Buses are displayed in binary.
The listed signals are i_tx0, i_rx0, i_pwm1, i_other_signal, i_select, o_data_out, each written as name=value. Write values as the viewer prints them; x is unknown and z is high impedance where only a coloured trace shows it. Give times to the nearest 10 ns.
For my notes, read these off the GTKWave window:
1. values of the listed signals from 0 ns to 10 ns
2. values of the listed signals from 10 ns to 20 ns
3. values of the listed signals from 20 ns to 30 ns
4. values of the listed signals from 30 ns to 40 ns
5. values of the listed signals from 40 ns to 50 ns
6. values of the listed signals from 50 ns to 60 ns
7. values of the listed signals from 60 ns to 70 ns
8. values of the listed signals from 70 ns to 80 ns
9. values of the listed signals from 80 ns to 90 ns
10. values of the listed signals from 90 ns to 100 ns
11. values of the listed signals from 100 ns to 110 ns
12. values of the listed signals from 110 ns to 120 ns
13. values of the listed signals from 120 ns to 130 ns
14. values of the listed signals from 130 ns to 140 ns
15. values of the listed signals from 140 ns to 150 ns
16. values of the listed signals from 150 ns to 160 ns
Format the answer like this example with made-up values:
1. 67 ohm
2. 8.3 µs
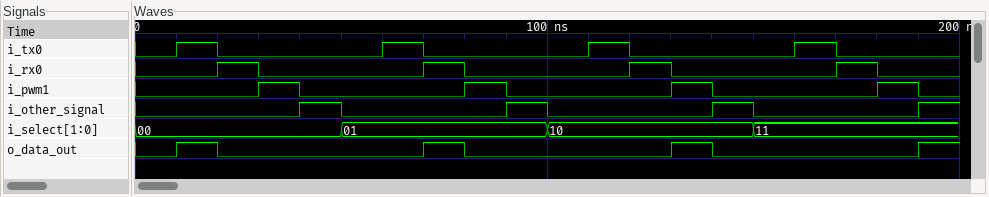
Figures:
1. i_tx0=0, i_rx0=0, i_pwm1=0, i_other_signal=0, i_select=00, o_data_out=0
2. i_tx0=1, i_rx0=0, i_pwm1=0, i_other_signal=0, i_select=00, o_data_out=1
3. i_tx0=0, i_rx0=1, i_pwm1=0, i_other_signal=0, i_select=00, o_data_out=0
4. i_tx0=0, i_rx0=0, i_pwm1=1, i_other_signal=0, i_select=00, o_data_out=0
5. i_tx0=0, i_rx0=0, i_pwm1=0, i_other_signal=1, i_select=00, o_data_out=0
6. i_tx0=0, i_rx0=0, i_pwm1=0, i_other_signal=0, i_select=01, o_data_out=0
7. i_tx0=1, i_rx0=0, i_pwm1=0, i_other_signal=0, i_select=01, o_data_out=0
8. i_tx0=0, i_rx0=1, i_pwm1=0, i_other_signal=0, i_select=01, o_data_out=1
9. i_tx0=0, i_rx0=0, i_pwm1=1, i_other_signal=0, i_select=01, o_data_out=0
10. i_tx0=0, i_rx0=0, i_pwm1=0, i_other_signal=1, i_select=01, o_data_out=0
11. i_tx0=0, i_rx0=0, i_pwm1=0, i_other_signal=0, i_select=10, o_data_out=0
12. i_tx0=1, i_rx0=0, i_pwm1=0, i_other_signal=0, i_select=10, o_data_out=0
13. i_tx0=0, i_rx0=1, i_pwm1=0, i_other_signal=0, i_select=10, o_data_out=0
14. i_tx0=0, i_rx0=0, i_pwm1=1, i_other_signal=0, i_select=10, o_data_out=1
15. i_tx0=0, i_rx0=0, i_pwm1=0, i_other_signal=1, i_select=10, o_data_out=0
16. i_tx0=0, i_rx0=0, i_pwm1=0, i_other_signal=0, i_select=11, o_data_out=0
